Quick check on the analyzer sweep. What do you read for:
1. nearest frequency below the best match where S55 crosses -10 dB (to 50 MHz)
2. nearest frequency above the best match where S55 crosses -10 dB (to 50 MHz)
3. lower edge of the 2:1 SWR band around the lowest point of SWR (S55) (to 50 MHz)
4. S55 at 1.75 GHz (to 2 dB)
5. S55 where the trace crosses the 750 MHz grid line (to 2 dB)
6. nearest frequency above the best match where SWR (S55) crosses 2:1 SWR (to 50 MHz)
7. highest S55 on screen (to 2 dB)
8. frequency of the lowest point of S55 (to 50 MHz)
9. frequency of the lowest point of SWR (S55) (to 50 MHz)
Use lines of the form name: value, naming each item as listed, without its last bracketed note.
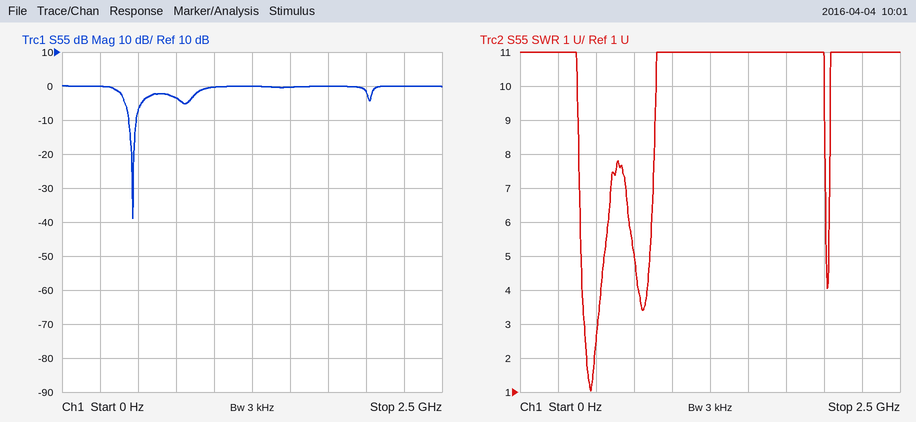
nearest frequency below the best match where S55 crosses -10 dB: 450 MHz
nearest frequency above the best match where S55 crosses -10 dB: 500 MHz
lower edge of the 2:1 SWR band around the lowest point of SWR (S55): 450 MHz
S55 at 1.75 GHz: 0 dB
S55 where the trace crosses the 750 MHz grid line: -4 dB
nearest frequency above the best match where SWR (S55) crosses 2:1 SWR: 500 MHz
highest S55 on screen: 0 dB
frequency of the lowest point of S55: 450 MHz
frequency of the lowest point of SWR (S55): 450 MHz
